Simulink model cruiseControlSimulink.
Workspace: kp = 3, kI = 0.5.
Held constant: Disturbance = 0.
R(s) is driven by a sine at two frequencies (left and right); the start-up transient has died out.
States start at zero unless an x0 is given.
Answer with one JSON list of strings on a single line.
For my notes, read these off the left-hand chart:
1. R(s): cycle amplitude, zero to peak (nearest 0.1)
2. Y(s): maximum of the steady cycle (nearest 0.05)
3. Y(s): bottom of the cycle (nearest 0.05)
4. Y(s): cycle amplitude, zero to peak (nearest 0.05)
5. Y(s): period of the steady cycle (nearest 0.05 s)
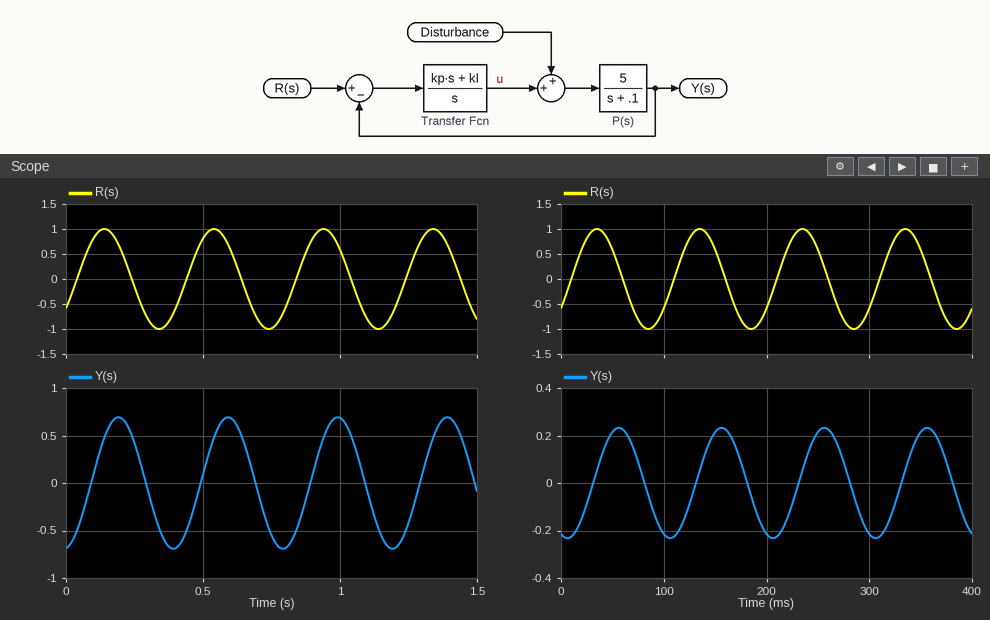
["1.0", "0.70", "-0.70", "0.70", "0.40 s"]
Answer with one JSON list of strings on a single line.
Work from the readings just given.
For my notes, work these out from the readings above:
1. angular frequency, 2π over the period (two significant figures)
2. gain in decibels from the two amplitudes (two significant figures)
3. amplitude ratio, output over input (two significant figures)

["16 rad/s", "-3.1 dB", "0.70"]
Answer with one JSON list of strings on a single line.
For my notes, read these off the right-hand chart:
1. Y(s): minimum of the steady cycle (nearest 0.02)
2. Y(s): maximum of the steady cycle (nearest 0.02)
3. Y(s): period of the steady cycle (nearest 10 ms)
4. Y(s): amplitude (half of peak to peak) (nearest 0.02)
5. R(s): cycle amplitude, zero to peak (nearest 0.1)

["-0.24", "0.24", "100 ms", "0.24", "1.0"]
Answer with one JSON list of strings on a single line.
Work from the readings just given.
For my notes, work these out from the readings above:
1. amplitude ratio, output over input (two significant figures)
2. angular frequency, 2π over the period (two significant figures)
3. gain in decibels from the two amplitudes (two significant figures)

["0.24", "0.063 rad/ms", "-12 dB"]
